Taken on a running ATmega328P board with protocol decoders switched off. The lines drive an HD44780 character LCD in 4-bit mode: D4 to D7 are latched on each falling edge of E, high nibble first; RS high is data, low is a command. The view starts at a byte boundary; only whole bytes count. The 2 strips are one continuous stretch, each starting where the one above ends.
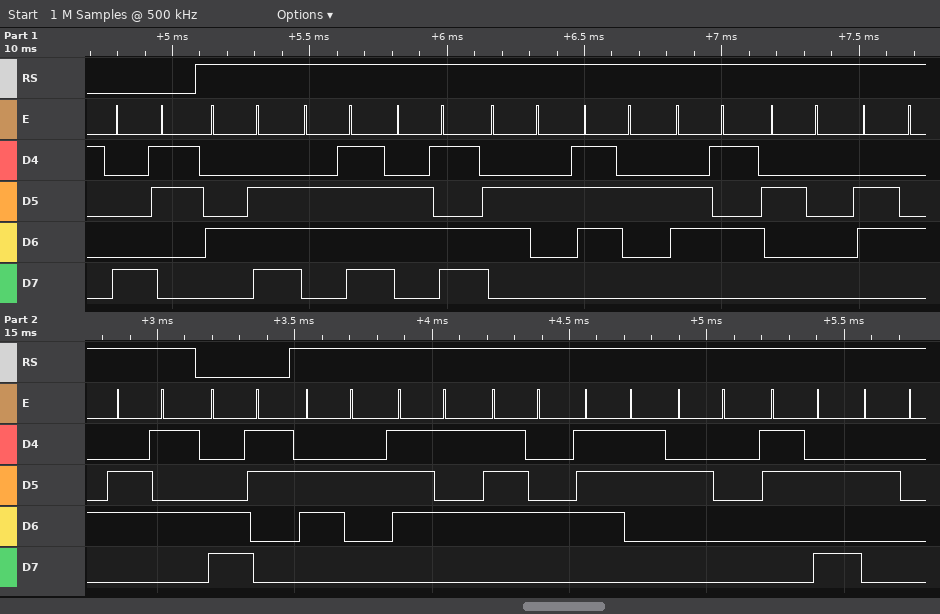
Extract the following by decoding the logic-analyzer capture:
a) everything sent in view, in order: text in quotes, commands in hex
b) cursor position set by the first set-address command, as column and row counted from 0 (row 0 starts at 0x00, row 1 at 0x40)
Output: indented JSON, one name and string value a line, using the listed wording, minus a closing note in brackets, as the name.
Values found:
{
  "everything sent in view, in order: text in quotes, commands in hex": "0x83 \"Nombre de\" 0xC3 \"buts : \"",
  "cursor position set by the first set-address command, as column and row counted from 0": "column 3, row 0"
}
